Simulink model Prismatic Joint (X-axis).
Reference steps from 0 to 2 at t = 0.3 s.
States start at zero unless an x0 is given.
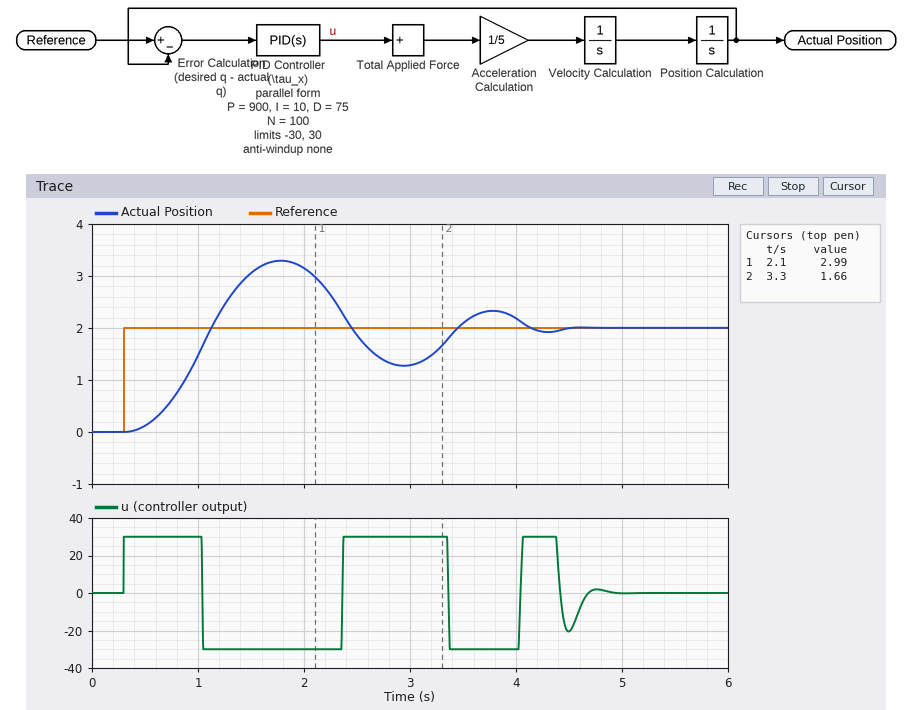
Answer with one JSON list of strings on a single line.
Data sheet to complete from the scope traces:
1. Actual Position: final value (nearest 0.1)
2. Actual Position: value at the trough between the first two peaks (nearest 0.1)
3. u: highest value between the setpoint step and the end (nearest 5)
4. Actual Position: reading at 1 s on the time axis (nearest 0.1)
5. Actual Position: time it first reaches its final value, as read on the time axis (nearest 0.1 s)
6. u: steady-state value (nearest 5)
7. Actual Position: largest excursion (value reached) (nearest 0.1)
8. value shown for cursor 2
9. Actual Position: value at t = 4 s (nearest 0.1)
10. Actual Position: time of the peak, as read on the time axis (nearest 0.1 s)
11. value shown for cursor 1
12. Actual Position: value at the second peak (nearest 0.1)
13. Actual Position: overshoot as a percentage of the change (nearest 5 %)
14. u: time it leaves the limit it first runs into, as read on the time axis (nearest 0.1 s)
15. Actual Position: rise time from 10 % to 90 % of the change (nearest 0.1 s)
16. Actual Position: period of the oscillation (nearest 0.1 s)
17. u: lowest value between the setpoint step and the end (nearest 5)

["2.0", "1.3", "30", "1.5", "1.1 s", "0", "3.3", "1.66", "2.2", "1.8 s", "2.99", "2.3", "65 %", "1.0 s", "0.5 s", "2.0 s", "-30"]
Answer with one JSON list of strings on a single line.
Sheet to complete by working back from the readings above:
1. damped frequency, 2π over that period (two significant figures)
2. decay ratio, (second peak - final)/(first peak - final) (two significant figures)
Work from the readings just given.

["3.1 rad/s", "0.23"]
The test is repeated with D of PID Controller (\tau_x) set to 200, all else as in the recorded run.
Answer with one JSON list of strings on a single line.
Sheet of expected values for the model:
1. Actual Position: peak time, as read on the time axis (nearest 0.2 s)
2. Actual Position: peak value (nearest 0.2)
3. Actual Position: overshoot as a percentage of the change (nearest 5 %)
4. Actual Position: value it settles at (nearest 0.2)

["1.6 s", "2.4", "20 %", "2.0"]
